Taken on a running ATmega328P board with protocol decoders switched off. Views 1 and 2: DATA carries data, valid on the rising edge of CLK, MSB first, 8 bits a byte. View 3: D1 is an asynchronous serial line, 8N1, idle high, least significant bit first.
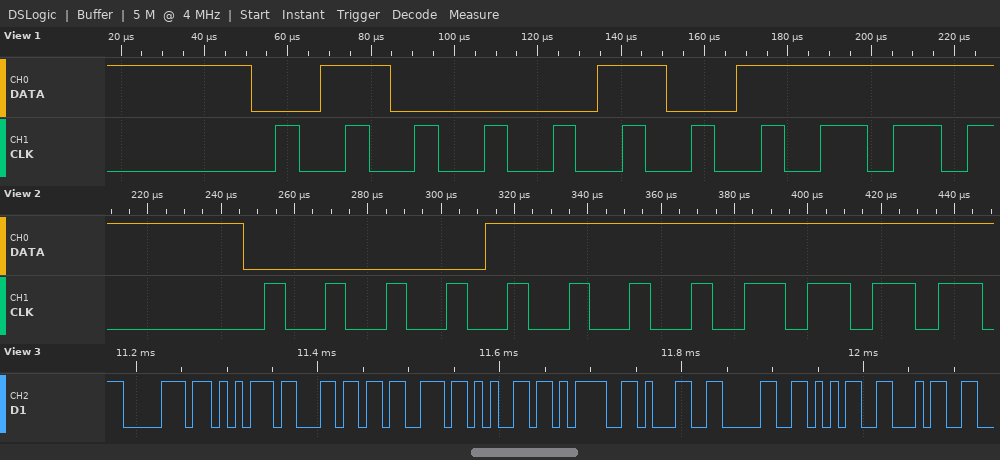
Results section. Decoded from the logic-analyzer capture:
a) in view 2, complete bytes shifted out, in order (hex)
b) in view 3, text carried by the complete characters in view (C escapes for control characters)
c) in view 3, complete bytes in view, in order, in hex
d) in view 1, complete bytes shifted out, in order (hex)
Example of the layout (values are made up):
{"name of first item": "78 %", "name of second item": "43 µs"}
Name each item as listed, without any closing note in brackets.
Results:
{"in view 2, complete bytes shifted out, in order": "0F", "in view 3, text carried by the complete characters in view": "\"pulse=1054\"", "in view 3, complete bytes in view, in order, in hex": "70 75 6C 73 65 3D 31 30 35 34", "in view 1, complete bytes shifted out, in order": "0x45"}
